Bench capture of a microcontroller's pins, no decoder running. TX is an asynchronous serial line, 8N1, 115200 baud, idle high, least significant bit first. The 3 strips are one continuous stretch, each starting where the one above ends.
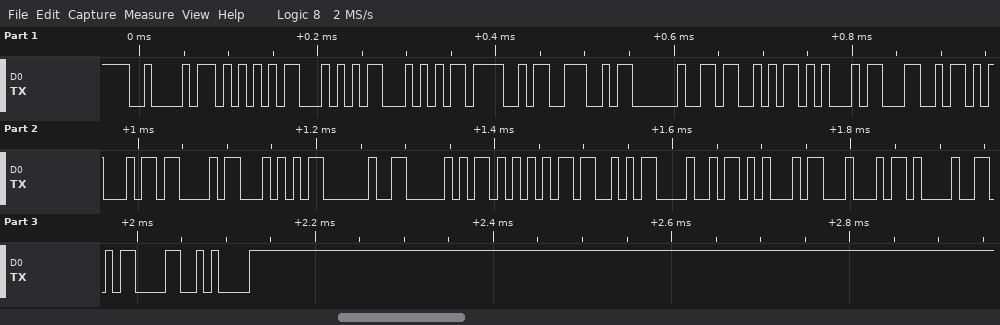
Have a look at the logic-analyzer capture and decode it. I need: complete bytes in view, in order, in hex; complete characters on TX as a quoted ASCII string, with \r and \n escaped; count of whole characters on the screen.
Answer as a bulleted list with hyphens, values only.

- 42 55 54 54 4F 4E 20 53 45 4C 45 43 54 20 50 55 53 48 45 44 21 0D 0A
- "BUTTON SELECT PUSHED!\r\n"
- 23
